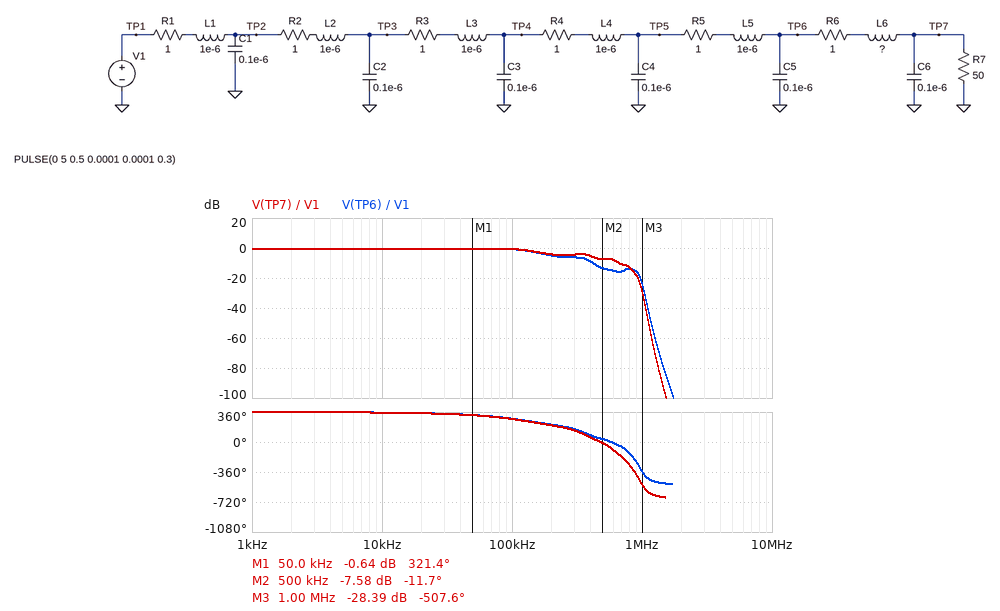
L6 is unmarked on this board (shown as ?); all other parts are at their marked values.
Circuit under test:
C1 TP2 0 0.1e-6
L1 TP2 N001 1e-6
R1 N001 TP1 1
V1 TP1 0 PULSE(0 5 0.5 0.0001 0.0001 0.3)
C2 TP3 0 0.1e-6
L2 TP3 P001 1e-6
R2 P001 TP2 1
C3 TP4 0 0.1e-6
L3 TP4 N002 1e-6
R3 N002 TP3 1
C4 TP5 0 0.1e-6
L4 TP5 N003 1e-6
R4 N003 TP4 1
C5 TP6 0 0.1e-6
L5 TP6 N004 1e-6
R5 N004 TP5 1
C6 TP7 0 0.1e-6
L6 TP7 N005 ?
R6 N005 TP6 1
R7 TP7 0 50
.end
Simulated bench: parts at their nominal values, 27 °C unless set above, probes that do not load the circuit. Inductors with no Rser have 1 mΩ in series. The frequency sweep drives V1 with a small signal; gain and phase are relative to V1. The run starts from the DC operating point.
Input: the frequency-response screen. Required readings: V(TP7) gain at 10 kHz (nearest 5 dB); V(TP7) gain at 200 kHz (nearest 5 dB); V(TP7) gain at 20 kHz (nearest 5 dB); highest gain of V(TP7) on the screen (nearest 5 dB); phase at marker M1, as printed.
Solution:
0 dB
-5 dB
0 dB
0 dB
321.4 deg
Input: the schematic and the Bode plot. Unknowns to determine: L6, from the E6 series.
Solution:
680 nH
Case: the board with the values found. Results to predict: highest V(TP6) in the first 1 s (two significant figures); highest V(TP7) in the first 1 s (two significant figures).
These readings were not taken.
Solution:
4.6 V
4.5 V
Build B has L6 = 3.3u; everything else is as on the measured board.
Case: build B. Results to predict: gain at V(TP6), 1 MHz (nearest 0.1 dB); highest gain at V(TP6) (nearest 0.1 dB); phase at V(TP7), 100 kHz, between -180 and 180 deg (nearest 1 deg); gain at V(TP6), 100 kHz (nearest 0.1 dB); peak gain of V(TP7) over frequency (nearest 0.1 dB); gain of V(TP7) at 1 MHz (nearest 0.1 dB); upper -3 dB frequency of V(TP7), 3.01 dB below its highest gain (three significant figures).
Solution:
-27.3 dB
-0.5 dB
-87 deg
-1.1 dB
0.7 dB
-48.9 dB
347 kHz
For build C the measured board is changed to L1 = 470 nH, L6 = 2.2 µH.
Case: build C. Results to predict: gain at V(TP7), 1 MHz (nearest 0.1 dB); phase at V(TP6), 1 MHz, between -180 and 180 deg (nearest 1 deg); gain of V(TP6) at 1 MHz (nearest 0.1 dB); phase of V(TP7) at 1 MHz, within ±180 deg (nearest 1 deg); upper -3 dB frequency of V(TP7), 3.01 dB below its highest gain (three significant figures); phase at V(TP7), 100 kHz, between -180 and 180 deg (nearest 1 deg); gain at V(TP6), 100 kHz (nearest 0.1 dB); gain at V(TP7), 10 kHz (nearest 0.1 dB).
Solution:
-36.1 dB
4 deg
-18.3 dB
-169 deg
430 kHz
-81 deg
-1.3 dB
-1.0 dB
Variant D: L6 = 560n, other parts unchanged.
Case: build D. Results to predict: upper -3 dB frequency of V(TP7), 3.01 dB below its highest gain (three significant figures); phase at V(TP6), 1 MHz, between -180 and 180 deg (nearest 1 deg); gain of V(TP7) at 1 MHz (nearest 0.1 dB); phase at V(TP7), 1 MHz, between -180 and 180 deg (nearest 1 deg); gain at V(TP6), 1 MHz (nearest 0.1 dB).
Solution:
175 kHz
29 deg
-28.5 dB
-120 deg
-25.7 dB
